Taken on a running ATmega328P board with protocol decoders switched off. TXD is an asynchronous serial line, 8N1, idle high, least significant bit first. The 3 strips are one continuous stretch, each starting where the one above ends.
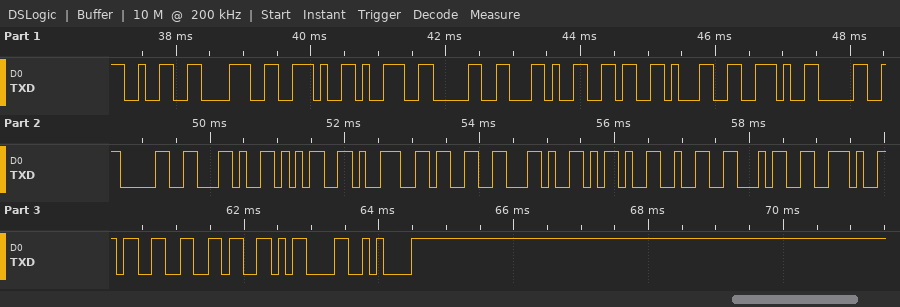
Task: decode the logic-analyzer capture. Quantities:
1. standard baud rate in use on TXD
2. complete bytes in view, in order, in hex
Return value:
9600 baud
32 38 2E 39 30 2C 36 31 2E 30 30 2C 35 39 33 2C 2D 32 34 2E 33 36 0D 0A
